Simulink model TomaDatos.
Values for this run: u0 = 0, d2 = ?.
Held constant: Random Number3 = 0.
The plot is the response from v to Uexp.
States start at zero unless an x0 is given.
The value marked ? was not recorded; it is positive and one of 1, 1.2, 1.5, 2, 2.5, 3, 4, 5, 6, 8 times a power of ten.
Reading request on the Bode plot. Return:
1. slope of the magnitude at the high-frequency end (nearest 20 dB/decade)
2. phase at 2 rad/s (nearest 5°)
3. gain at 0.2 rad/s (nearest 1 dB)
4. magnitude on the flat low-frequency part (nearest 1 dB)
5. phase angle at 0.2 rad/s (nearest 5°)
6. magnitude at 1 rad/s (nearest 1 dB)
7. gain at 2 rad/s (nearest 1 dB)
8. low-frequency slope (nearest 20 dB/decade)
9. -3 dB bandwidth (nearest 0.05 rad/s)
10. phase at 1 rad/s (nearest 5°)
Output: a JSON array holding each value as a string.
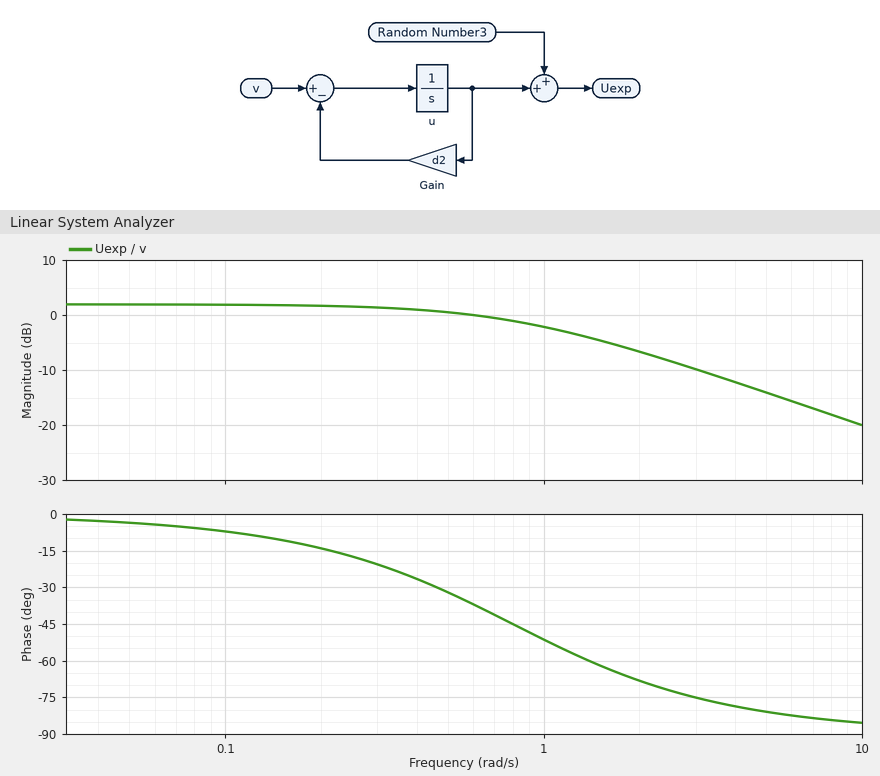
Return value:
["-20 dB/decade", "-70°", "2 dB", "2 dB", "-15°", "-2 dB", "-7 dB", "0 dB/decade", "0.80 rad/s", "-50°"]
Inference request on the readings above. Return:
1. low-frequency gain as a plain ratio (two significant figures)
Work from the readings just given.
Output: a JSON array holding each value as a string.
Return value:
["1.3"]
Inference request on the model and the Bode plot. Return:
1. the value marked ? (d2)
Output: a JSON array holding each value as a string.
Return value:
["0.8"]
